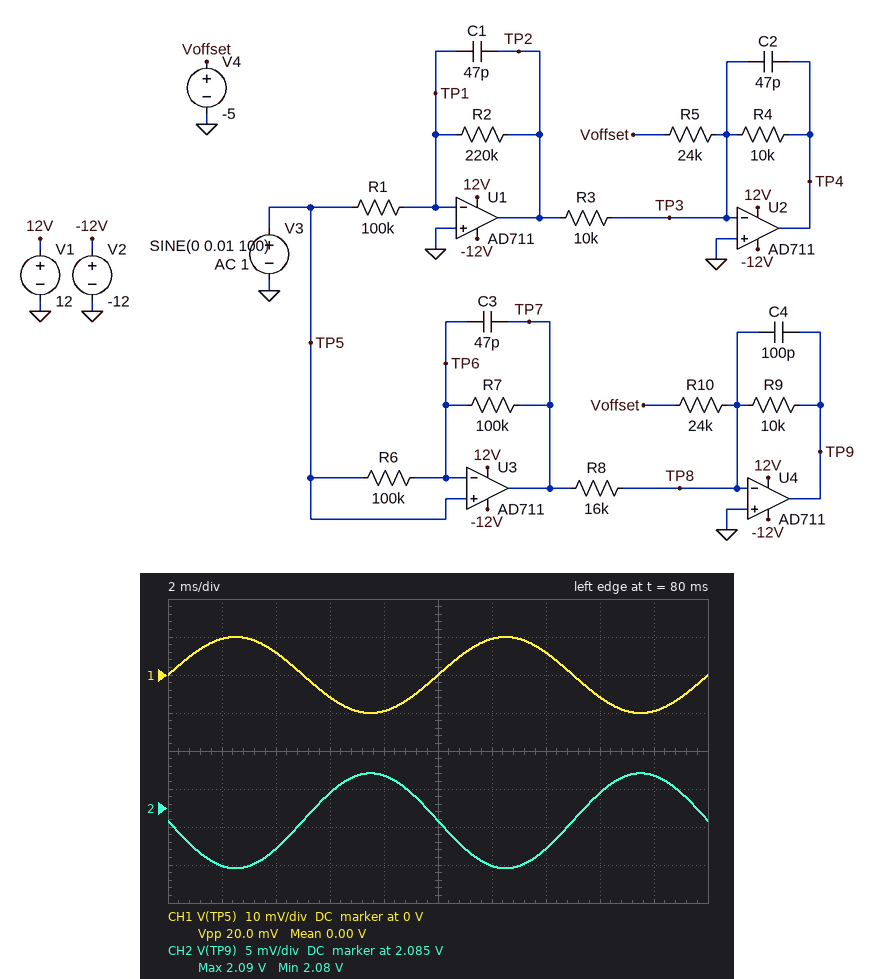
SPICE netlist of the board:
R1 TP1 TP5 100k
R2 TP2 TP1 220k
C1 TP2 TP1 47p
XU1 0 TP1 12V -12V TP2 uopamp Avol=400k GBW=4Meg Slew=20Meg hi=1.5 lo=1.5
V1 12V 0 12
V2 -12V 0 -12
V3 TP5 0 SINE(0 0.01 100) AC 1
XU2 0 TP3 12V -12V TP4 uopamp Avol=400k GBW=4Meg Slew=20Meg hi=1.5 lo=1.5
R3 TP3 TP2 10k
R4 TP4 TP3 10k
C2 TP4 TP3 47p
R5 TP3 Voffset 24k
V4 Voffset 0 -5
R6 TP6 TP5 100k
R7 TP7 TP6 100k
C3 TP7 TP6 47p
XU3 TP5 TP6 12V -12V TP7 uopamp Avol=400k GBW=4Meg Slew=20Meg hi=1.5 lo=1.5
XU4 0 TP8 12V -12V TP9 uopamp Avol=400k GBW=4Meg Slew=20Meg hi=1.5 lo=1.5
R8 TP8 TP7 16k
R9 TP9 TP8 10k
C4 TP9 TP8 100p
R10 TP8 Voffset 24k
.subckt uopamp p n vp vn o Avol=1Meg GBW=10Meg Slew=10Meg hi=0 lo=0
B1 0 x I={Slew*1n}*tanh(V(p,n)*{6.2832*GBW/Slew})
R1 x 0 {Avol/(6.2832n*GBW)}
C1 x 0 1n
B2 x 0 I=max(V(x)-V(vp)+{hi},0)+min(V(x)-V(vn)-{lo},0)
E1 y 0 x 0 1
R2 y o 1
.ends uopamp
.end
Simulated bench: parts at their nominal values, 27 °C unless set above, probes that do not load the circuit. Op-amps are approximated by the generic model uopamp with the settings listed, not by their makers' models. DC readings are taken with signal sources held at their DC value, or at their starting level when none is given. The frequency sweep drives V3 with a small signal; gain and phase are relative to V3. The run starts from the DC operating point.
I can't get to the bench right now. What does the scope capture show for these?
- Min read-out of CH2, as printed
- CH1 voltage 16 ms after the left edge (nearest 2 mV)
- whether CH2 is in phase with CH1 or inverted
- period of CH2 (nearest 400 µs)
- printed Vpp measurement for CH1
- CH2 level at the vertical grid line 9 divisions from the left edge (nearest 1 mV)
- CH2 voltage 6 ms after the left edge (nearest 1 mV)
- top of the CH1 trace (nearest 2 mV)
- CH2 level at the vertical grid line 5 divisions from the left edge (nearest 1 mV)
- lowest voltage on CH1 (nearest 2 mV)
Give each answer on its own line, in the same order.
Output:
2.08 V
-6 mV
inverted
10.0 ms
20.0 mV
2.089 V
2.087 V
10 mV
2.083 V
-10 mV
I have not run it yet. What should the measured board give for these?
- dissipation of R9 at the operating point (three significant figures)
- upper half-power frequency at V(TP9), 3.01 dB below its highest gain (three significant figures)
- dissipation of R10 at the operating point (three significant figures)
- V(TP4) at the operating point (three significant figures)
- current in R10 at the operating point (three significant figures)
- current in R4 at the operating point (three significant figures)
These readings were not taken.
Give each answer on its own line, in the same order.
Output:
434 µW
150 kHz
1.04 mW
2.08 V
208 µA
208 µA
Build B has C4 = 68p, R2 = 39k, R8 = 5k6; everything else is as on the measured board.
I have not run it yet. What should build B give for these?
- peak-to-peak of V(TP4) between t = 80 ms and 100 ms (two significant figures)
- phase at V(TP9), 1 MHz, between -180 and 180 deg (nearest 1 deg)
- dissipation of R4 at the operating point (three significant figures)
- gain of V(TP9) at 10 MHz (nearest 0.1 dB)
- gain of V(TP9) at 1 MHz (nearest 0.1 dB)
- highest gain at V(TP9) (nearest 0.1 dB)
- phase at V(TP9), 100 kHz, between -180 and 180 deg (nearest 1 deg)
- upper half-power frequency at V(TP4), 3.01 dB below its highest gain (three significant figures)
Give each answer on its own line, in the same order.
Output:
7.8 mV
75 deg
434 µW
-44.9 dB
-9.4 dB
5.0 dB
151 deg
80.1 kHz
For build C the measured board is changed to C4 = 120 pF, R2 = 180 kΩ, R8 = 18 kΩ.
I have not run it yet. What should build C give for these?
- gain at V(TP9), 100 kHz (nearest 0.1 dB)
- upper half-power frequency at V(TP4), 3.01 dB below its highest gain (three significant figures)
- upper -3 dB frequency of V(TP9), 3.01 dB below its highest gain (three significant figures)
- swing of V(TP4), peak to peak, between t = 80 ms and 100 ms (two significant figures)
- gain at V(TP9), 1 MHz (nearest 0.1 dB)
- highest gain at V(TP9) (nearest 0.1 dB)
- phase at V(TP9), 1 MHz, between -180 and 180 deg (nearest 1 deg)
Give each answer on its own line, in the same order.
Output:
-7.2 dB
18.6 kHz
126 kHz
36 mV
-23.6 dB
-5.1 dB
70 deg
